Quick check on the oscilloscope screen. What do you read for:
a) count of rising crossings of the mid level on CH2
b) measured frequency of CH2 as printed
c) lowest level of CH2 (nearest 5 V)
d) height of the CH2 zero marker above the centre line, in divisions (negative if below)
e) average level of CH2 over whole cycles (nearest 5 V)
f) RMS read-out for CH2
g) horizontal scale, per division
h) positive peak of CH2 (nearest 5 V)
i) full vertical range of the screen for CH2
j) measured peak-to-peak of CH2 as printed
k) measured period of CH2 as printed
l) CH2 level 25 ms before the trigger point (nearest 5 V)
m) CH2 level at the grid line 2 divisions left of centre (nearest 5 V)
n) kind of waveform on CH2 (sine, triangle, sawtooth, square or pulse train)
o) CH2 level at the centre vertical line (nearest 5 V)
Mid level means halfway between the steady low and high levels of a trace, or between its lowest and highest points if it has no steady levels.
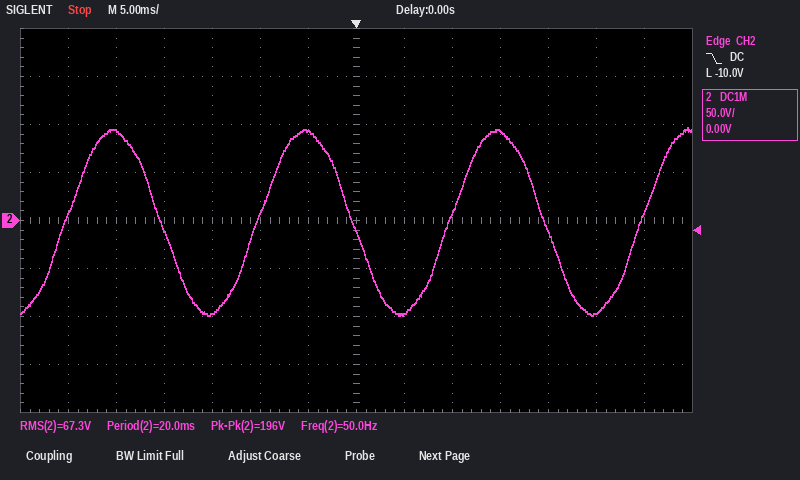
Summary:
4
50.0 Hz
-100 V
0.0 div
0 V
67.3 V
5 ms
95 V
400 V
196 V
20.0 ms
95 V
5 V
sine
-10 V
